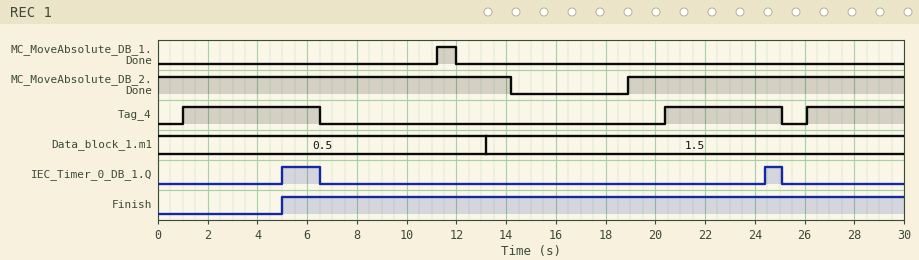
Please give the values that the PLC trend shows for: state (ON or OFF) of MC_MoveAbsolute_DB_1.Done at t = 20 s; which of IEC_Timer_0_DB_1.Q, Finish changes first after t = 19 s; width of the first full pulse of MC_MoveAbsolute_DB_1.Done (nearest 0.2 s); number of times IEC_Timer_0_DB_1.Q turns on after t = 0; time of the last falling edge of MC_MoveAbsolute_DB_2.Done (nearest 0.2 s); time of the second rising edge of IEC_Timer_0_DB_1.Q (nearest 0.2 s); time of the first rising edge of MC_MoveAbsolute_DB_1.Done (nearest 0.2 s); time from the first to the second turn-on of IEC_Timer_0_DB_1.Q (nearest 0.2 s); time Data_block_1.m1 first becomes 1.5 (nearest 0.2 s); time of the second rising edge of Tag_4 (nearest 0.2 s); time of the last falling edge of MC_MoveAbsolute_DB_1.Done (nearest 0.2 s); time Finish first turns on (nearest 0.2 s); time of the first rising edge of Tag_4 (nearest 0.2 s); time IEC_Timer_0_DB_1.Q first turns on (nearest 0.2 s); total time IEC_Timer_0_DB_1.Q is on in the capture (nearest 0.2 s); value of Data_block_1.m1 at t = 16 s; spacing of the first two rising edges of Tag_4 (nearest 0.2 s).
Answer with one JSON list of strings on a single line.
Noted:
["OFF", "IEC_Timer_0_DB_1.Q", "0.8 s", "2", "14.2 s", "24.4 s", "11.2 s", "19.4 s", "13.2 s", "20.4 s", "12.0 s", "5.0 s", "1.0 s", "5.0 s", "2.2 s", "1.5", "19.4 s"]
